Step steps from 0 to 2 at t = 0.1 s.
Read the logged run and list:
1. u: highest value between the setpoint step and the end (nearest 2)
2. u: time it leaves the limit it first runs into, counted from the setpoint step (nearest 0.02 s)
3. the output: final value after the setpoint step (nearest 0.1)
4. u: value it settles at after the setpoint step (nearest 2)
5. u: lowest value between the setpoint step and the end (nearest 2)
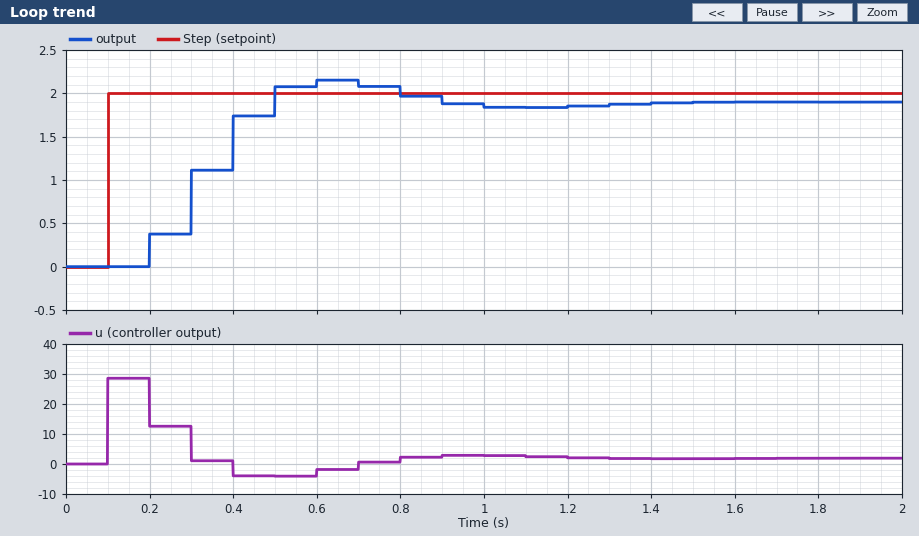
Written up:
28
0.10 s
1.9
2
-4
